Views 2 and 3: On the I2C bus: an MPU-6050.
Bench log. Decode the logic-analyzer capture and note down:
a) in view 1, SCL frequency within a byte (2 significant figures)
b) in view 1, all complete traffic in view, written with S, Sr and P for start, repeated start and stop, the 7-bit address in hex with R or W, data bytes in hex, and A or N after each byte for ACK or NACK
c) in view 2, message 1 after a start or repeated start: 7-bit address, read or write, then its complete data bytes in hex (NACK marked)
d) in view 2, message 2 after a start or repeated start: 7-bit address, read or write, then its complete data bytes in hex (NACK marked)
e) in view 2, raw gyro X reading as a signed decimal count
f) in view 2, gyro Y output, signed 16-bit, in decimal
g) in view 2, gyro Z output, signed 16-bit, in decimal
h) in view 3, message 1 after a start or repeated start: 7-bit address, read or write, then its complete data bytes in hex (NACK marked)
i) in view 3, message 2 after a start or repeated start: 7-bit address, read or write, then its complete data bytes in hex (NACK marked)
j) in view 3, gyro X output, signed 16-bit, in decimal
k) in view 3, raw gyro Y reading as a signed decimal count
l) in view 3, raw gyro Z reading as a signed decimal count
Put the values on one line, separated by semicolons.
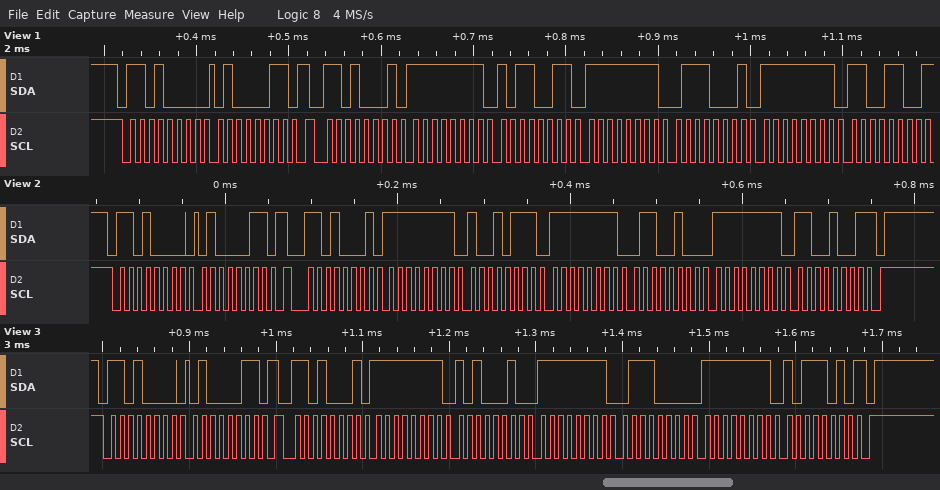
100 kHz; S 68W A 43 A Sr 68R A FF A B3 A FF A 71 A FF A CC N; 0x68 write: 43; 0x68 read: FF 97 FF 64 FF C9 NACK; -105; -156; -55; 0x68 write: 43; 0x68 read: FF A2 FF 70 FF BA NACK; -94; -144; -70
